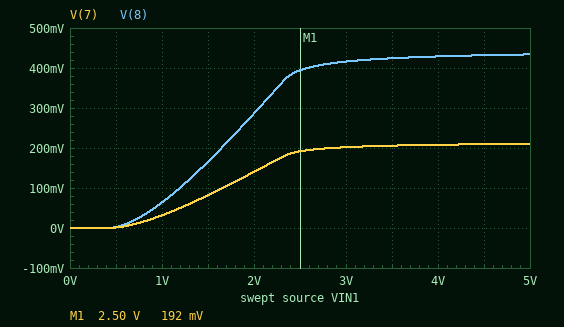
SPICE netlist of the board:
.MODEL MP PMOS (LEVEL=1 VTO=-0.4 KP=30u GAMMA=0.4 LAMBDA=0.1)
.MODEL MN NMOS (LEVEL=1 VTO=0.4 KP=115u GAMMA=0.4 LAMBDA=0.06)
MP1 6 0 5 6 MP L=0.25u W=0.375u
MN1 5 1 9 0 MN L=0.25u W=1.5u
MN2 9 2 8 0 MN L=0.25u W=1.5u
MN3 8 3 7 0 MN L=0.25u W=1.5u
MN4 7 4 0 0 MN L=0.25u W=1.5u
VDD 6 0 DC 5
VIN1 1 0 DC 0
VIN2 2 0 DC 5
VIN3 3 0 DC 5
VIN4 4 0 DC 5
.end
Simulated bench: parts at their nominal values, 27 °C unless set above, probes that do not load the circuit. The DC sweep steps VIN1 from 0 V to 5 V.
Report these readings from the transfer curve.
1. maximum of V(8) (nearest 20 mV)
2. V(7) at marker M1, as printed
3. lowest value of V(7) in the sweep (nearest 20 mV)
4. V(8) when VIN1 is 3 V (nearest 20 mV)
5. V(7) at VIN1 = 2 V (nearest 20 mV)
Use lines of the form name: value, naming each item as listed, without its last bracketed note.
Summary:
maximum of V(8): 440 mV
V(7) at marker M1, as printed: 192 mV
lowest value of V(7) in the sweep: 0 V
V(8) when VIN1 is 3 V: 420 mV
V(7) at VIN1 = 2 V: 140 mV
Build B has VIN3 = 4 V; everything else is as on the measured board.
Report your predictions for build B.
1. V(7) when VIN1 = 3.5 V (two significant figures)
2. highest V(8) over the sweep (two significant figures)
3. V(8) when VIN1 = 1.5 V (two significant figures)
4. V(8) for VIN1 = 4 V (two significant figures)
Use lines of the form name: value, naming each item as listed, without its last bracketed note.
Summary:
V(7) when VIN1 = 3.5 V: 200 mV
highest V(8) over the sweep: 500 mV
V(8) when VIN1 = 1.5 V: 180 mV
V(8) for VIN1 = 4 V: 490 mV
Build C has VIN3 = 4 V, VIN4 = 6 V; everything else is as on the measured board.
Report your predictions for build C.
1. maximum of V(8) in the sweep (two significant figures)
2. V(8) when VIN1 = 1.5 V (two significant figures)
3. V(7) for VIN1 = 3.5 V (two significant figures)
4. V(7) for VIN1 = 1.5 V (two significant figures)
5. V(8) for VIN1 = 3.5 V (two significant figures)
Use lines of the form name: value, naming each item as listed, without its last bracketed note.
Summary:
maximum of V(8) in the sweep: 460 mV
V(8) when VIN1 = 1.5 V: 170 mV
V(7) for VIN1 = 3.5 V: 170 mV
V(7) for VIN1 = 1.5 V: 66 mV
V(8) for VIN1 = 3.5 V: 450 mV
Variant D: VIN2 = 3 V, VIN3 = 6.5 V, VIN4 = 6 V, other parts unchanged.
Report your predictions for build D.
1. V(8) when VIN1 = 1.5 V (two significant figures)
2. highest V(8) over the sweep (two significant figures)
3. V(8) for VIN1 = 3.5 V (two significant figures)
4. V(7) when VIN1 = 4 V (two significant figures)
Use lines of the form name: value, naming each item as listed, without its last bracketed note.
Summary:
V(8) when VIN1 = 1.5 V: 120 mV
highest V(8) over the sweep: 330 mV
V(8) for VIN1 = 3.5 V: 320 mV
V(7) when VIN1 = 4 V: 170 mV
